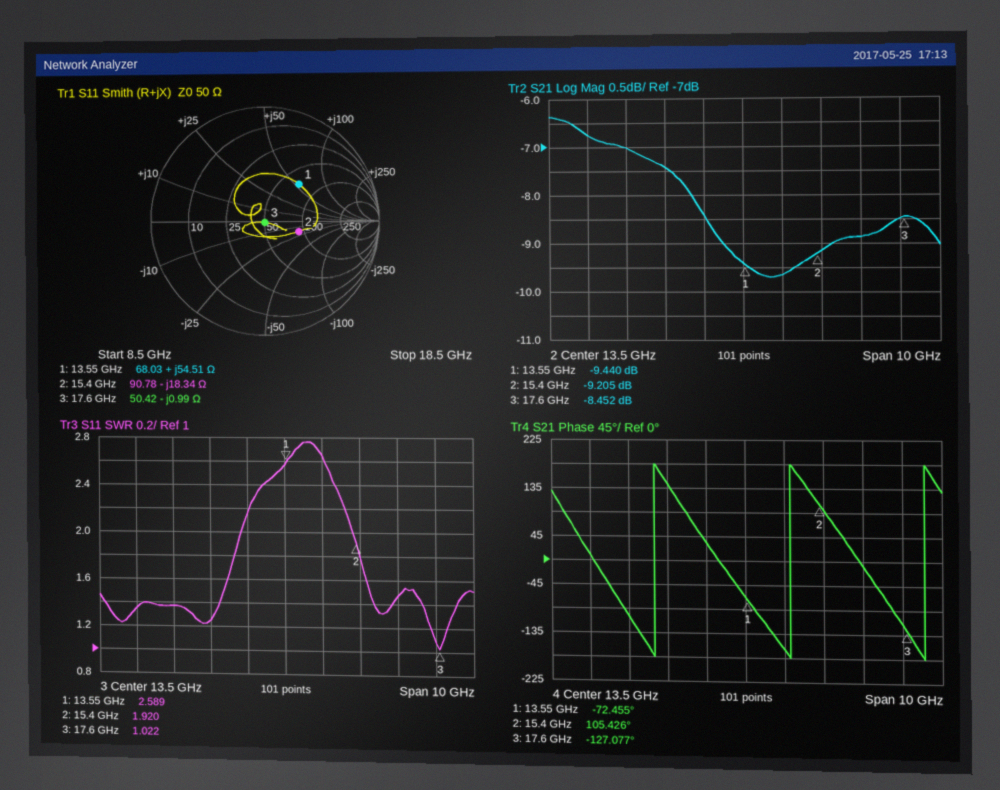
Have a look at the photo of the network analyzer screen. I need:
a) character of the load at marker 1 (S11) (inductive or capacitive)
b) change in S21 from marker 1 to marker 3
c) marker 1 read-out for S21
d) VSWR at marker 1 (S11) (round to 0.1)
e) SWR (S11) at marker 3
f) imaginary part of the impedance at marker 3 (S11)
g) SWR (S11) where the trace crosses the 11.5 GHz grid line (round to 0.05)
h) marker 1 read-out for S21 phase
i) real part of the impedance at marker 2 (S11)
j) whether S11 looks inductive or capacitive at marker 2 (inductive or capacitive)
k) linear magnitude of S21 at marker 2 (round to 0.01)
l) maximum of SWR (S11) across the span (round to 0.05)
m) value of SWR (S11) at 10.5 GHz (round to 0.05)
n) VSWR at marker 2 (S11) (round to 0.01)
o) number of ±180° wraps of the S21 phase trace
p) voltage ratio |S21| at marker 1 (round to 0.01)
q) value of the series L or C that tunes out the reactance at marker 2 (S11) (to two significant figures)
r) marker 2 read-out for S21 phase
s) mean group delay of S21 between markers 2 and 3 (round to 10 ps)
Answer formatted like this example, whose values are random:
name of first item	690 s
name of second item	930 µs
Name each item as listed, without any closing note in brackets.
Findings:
character of the load at marker 1 (S11)	inductive
change in S21 from marker 1 to marker 3	0.988 dB
marker 1 read-out for S21	-9.440 dB
VSWR at marker 1 (S11)	2.6
SWR (S11) at marker 3	1.022
imaginary part of the impedance at marker 3	-0.99 Ω
SWR (S11) where the trace crosses the 11.5 GHz grid line	1.25
marker 1 read-out for S21 phase	-72.455°
real part of the impedance at marker 2	90.78 Ω
whether S11 looks inductive or capacitive at marker 2	capacitive
linear magnitude of S21 at marker 2	0.35
maximum of SWR (S11) across the span	2.75
value of SWR (S11) at 10.5 GHz	1.35
VSWR at marker 2 (S11)	1.92
number of ±180° wraps of the S21 phase trace	3
voltage ratio |S21| at marker 1	0.34
value of the series L or C that tunes out the reactance at marker 2 (S11)	190 pH
marker 2 read-out for S21 phase	105.426°
mean group delay of S21 between markers 2 and 3	290 ps
